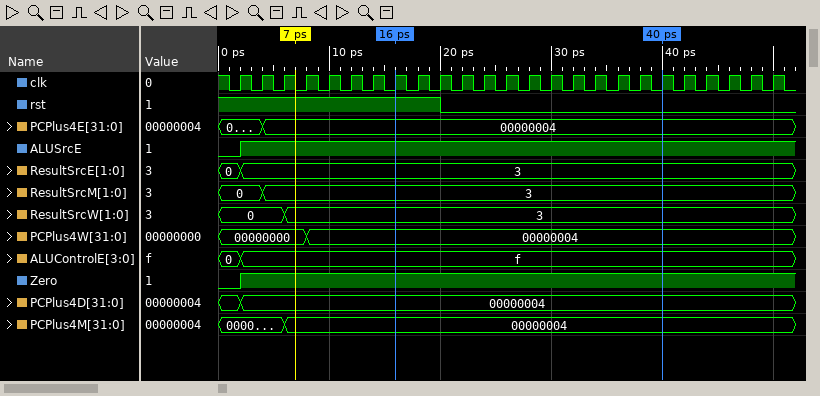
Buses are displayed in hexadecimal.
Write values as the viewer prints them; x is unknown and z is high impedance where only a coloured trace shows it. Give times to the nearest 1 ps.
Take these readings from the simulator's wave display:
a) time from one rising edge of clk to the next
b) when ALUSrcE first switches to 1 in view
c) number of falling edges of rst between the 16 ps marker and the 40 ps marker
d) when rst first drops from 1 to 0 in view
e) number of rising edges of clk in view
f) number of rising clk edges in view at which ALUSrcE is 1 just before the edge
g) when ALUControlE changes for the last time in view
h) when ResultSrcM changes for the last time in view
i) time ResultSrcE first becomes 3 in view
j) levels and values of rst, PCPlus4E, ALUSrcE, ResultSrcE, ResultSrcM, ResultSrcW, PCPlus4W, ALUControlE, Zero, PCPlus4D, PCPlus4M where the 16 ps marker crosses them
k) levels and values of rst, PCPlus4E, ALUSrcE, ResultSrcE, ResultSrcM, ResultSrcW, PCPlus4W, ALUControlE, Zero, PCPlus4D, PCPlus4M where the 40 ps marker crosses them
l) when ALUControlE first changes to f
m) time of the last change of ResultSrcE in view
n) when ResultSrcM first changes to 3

2 ps
2 ps
1
20 ps
25
24
2 ps
4 ps
2 ps
rst=1, PCPlus4E=00000004, ALUSrcE=1, ResultSrcE=3, ResultSrcM=3, ResultSrcW=3, PCPlus4W=00000004, ALUControlE=f, Zero=1, PCPlus4D=00000004, PCPlus4M=00000004
rst=0, PCPlus4E=00000004, ALUSrcE=1, ResultSrcE=3, ResultSrcM=3, ResultSrcW=3, PCPlus4W=00000004, ALUControlE=f, Zero=1, PCPlus4D=00000004, PCPlus4M=00000004
2 ps
2 ps
4 ps
